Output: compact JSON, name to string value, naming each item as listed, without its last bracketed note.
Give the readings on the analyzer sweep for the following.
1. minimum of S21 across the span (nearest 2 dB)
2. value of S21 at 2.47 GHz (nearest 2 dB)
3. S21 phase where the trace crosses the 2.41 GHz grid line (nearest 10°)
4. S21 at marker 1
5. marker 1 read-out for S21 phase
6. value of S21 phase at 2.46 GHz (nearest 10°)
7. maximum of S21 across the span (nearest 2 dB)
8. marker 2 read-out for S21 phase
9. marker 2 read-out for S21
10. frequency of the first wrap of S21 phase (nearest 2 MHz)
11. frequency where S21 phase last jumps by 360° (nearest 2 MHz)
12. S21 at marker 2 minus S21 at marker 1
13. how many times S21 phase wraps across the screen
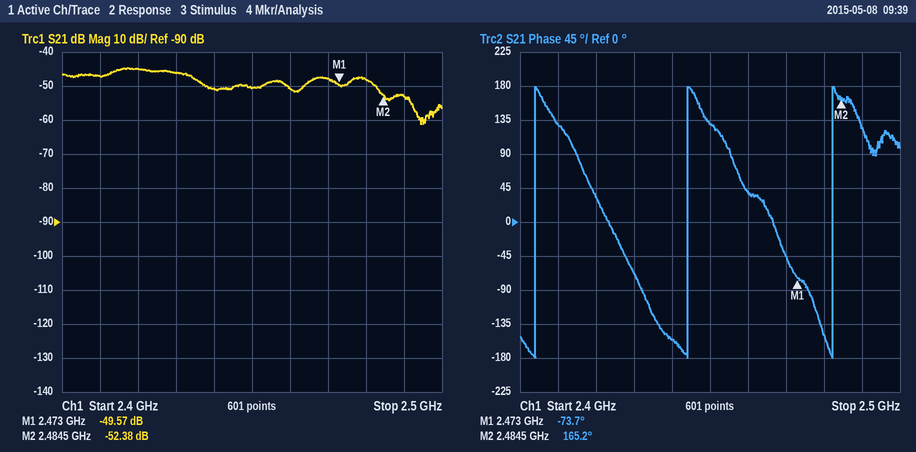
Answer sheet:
{"minimum of S21 across the span": "-62 dB", "value of S21 at 2.47 GHz": "-48 dB", "S21 phase where the trace crosses the 2.41 GHz grid line": "130°", "S21 at marker 1": "-49.57 dB", "marker 1 read-out for S21 phase": "-73.7°", "value of S21 phase at 2.46 GHz": "40°", "maximum of S21 across the span": "-44 dB", "marker 2 read-out for S21 phase": "165.2°", "marker 2 read-out for S21": "-52.38 dB", "frequency of the first wrap of S21 phase": "2.404 GHz", "frequency where S21 phase last jumps by 360°": "2.482 GHz", "S21 at marker 2 minus S21 at marker 1": "-2.81 dB", "how many times S21 phase wraps across the screen": "3"}
